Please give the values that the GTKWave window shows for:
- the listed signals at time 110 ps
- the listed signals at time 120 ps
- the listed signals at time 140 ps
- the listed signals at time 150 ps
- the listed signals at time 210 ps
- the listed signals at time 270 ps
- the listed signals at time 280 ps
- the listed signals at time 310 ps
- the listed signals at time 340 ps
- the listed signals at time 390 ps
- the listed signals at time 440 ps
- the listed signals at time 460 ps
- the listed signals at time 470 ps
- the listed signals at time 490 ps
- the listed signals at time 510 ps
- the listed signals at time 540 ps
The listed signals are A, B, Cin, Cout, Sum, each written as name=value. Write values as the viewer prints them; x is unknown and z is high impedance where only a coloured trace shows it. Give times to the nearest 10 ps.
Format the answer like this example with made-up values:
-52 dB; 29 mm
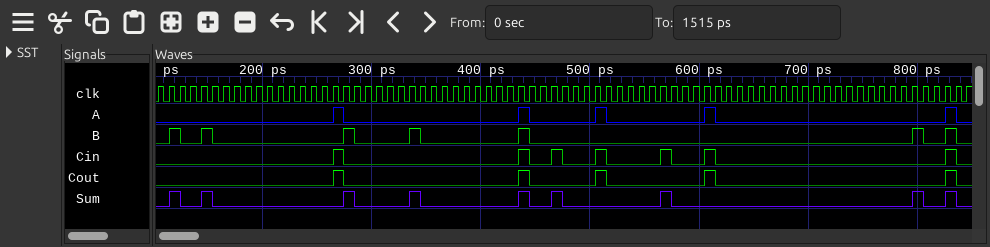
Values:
A=0, B=0, Cin=0, Cout=0, Sum=0; A=0, B=1, Cin=0, Cout=0, Sum=1; A=0, B=0, Cin=0, Cout=0, Sum=0; A=0, B=1, Cin=0, Cout=0, Sum=1; A=0, B=0, Cin=0, Cout=0, Sum=0; A=1, B=0, Cin=1, Cout=1, Sum=0; A=0, B=1, Cin=0, Cout=0, Sum=1; A=0, B=0, Cin=0, Cout=0, Sum=0; A=0, B=1, Cin=0, Cout=0, Sum=1; A=0, B=0, Cin=0, Cout=0, Sum=0; A=1, B=1, Cin=1, Cout=1, Sum=1; A=0, B=0, Cin=0, Cout=0, Sum=0; A=0, B=0, Cin=1, Cout=0, Sum=1; A=0, B=0, Cin=0, Cout=0, Sum=0; A=1, B=0, Cin=1, Cout=1, Sum=0; A=0, B=0, Cin=0, Cout=0, Sum=0
